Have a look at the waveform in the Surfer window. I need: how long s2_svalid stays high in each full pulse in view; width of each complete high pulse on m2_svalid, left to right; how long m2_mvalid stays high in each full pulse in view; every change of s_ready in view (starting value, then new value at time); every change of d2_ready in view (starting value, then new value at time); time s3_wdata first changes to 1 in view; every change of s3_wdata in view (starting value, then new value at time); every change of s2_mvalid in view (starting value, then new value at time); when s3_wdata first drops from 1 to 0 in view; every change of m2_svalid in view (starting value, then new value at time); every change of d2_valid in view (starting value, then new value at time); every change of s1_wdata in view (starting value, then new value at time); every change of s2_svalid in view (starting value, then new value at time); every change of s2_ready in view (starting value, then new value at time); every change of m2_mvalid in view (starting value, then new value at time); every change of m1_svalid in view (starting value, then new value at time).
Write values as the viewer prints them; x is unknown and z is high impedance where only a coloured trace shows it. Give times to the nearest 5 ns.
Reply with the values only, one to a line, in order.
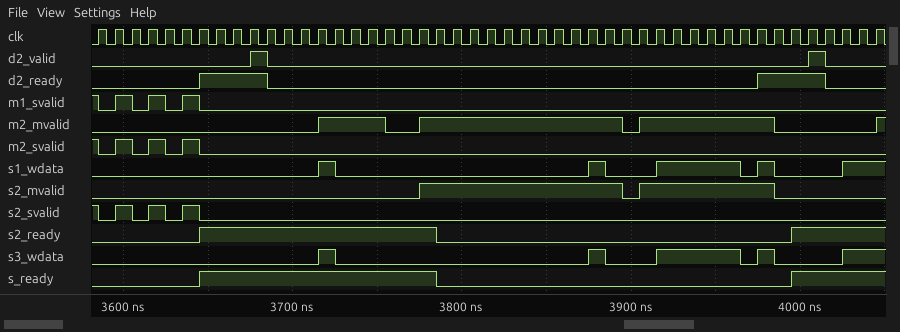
10 ns, 10 ns, 10 ns
10 ns, 10 ns, 10 ns
40 ns, 120 ns, 80 ns
0, 1 at 3645 ns, 0 at 3785 ns, 1 at 3995 ns
0, 1 at 3645 ns, 0 at 3685 ns, 1 at 3975 ns, 0 at 4015 ns
3715 ns
0, 1 at 3715 ns, 0 at 3725 ns, 1 at 3875 ns, 0 at 3885 ns, 1 at 3915 ns, 0 at 3965 ns, 1 at 3975 ns, 0 at 3985 ns, 1 at 4025 ns
0, 1 at 3775 ns, 0 at 3895 ns, 1 at 3905 ns, 0 at 3985 ns
3725 ns
1, 0 at 3585 ns, 1 at 3595 ns, 0 at 3605 ns, 1 at 3615 ns, 0 at 3625 ns, 1 at 3635 ns, 0 at 3645 ns
0, 1 at 3675 ns, 0 at 3685 ns, 1 at 4005 ns, 0 at 4015 ns
0, 1 at 3715 ns, 0 at 3725 ns, 1 at 3875 ns, 0 at 3885 ns, 1 at 3915 ns, 0 at 3965 ns, 1 at 3975 ns, 0 at 3985 ns, 1 at 4025 ns
1, 0 at 3585 ns, 1 at 3595 ns, 0 at 3605 ns, 1 at 3615 ns, 0 at 3625 ns, 1 at 3635 ns, 0 at 3645 ns
0, 1 at 3645 ns, 0 at 3785 ns, 1 at 3995 ns
0, 1 at 3715 ns, 0 at 3755 ns, 1 at 3775 ns, 0 at 3895 ns, 1 at 3905 ns, 0 at 3985 ns, 1 at 4045 ns
1, 0 at 3585 ns, 1 at 3595 ns, 0 at 3605 ns, 1 at 3615 ns, 0 at 3625 ns, 1 at 3635 ns, 0 at 3645 ns
